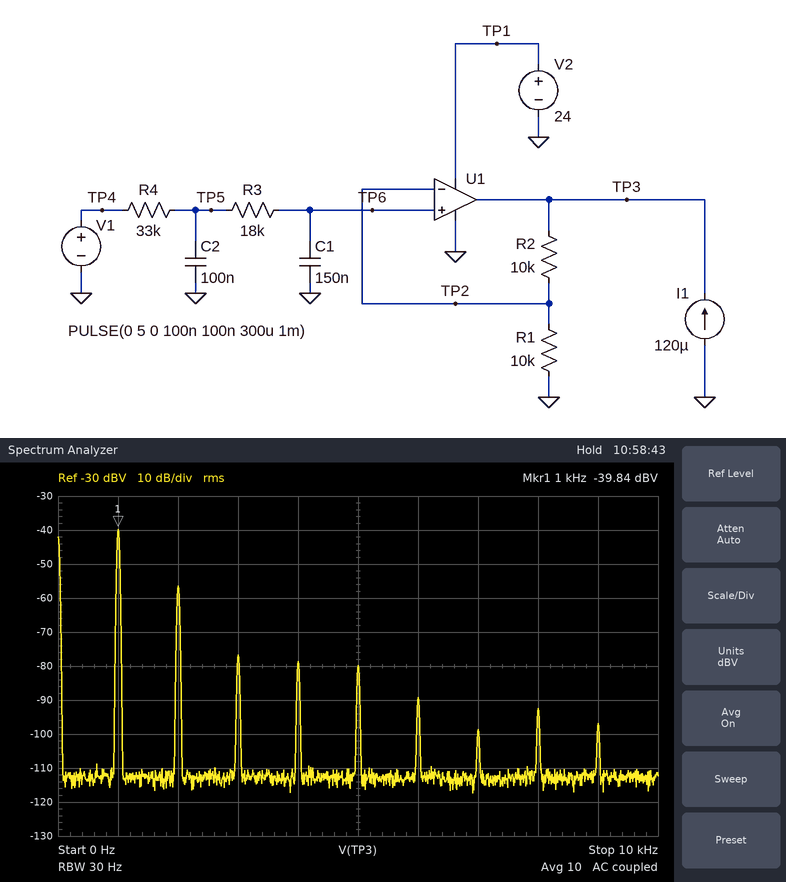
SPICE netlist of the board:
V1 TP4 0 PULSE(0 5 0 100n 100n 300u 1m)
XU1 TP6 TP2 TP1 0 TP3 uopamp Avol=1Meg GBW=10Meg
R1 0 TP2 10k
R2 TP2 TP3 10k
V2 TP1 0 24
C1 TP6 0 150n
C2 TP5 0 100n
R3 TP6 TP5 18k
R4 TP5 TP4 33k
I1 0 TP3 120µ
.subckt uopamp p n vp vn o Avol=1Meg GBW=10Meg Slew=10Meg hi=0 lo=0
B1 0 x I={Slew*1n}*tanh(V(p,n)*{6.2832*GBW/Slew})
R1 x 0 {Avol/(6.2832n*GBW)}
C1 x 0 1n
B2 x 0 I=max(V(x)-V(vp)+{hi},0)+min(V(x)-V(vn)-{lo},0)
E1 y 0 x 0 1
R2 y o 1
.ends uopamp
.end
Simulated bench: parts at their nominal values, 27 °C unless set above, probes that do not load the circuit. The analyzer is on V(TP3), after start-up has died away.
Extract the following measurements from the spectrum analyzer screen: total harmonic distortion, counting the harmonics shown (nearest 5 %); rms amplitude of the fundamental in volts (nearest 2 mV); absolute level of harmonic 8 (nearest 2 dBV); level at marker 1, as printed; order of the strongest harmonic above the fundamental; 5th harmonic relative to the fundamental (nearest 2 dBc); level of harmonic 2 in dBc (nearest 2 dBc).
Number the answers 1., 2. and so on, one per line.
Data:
1. 15 %
2. 10 mV
3. -92 dBV
4. -39.84 dBV
5. 2
6. -40 dBc
7. -16 dBc
